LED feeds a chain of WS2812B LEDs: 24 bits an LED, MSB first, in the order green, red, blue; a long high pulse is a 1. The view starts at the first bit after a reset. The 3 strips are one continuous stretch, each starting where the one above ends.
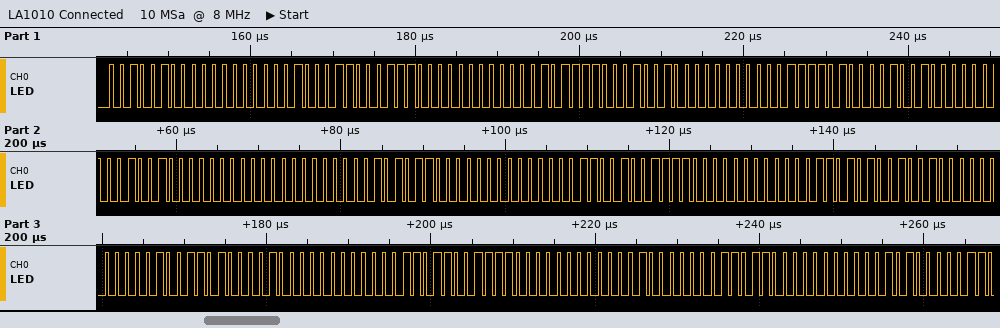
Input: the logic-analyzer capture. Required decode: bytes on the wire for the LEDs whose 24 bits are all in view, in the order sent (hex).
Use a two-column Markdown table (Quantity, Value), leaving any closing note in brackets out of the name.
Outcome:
| Quantity | Value |
|---|---|
| bytes on the wire for the LEDs whose 24 bits are all in view, in the order sent | 24 00 23 1C 00 2F 12 00 3D 09 00 48 00 00 56 00 06 4F 00 0D 49 00 13 42 00 1B 3C 00 20 36 |
